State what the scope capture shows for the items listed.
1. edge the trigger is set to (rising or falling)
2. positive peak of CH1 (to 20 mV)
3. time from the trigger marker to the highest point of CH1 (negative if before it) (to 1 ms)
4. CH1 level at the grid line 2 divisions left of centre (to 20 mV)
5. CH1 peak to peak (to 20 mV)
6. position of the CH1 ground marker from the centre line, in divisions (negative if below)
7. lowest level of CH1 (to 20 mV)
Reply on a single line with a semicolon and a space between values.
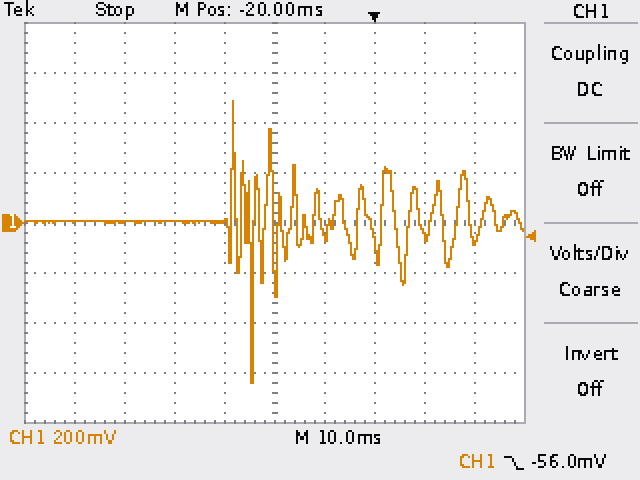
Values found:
falling; 480 mV; -28 ms; 0 mV; 1.12 V; 0.0 div; -640 mV
